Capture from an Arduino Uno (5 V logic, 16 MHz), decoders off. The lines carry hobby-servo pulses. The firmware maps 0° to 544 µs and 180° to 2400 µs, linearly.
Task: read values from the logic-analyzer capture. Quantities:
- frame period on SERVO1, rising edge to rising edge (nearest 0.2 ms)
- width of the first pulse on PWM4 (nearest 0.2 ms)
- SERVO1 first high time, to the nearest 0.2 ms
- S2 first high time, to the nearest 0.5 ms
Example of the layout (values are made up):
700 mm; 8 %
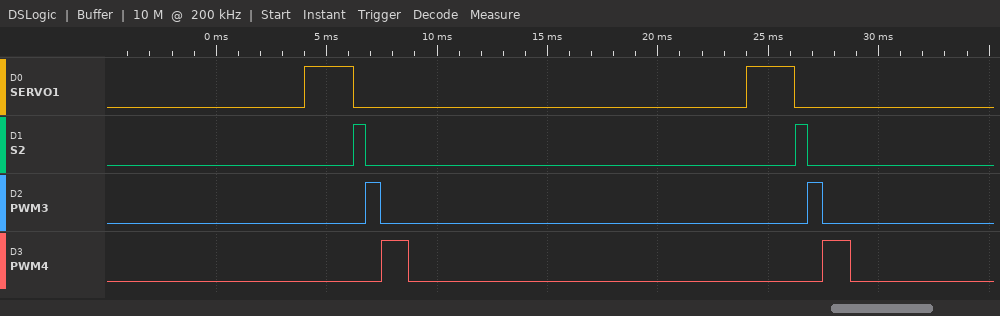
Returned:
20.0 ms; 1.2 ms; 2.2 ms; 0.5 ms
